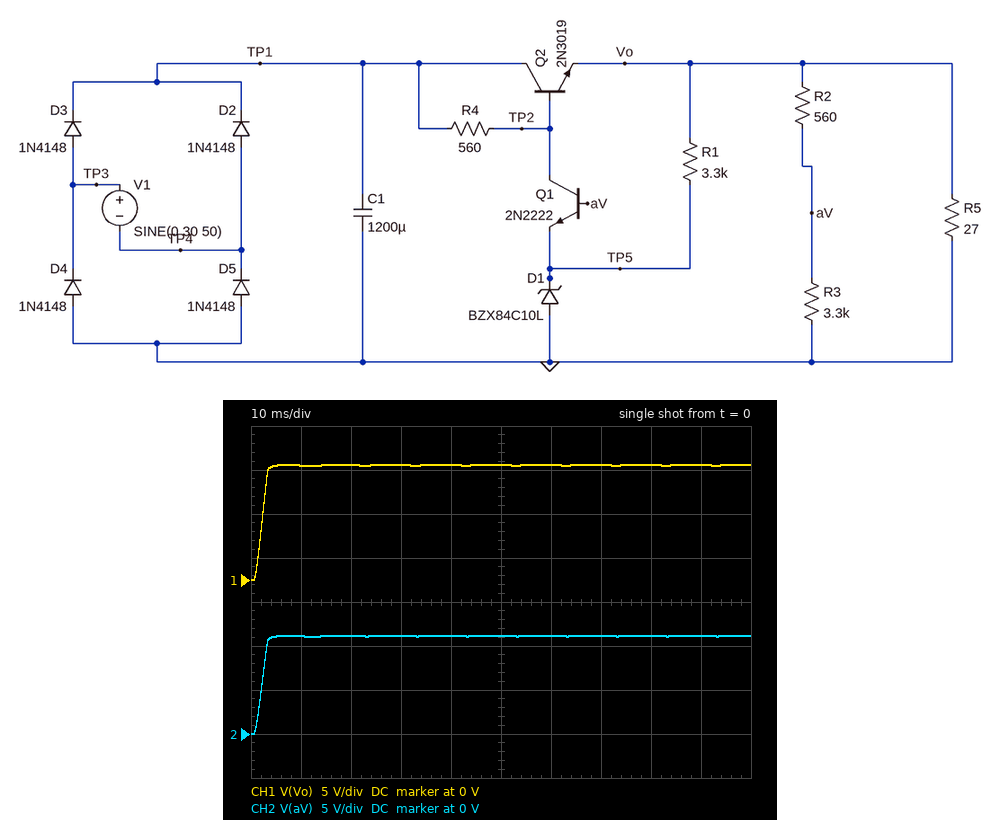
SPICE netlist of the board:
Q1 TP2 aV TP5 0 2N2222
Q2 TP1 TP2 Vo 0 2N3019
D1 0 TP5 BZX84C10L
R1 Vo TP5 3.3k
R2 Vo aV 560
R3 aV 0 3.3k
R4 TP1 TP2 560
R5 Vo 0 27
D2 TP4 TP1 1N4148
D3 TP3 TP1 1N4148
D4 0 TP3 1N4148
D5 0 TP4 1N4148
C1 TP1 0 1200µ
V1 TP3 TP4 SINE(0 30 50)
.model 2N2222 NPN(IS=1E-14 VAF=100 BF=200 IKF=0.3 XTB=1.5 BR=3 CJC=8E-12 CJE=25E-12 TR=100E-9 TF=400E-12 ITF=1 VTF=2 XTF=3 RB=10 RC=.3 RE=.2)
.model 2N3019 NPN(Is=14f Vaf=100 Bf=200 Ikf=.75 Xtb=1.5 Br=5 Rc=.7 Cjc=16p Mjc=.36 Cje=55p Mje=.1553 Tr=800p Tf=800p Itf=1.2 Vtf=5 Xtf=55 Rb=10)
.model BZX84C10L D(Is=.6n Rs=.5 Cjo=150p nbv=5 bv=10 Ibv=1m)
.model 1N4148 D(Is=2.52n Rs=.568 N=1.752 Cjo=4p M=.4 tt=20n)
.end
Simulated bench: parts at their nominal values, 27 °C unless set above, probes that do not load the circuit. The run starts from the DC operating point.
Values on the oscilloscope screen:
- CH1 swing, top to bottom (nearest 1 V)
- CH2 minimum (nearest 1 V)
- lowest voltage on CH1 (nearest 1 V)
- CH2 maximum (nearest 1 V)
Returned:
13 V
0 V
0 V
11 V
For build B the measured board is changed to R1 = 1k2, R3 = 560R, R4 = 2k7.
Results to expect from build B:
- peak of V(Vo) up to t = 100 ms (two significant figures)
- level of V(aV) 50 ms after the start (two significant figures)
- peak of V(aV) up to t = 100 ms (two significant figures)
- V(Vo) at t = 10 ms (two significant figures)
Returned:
14 V
6.8 V
7.2 V
13 V
